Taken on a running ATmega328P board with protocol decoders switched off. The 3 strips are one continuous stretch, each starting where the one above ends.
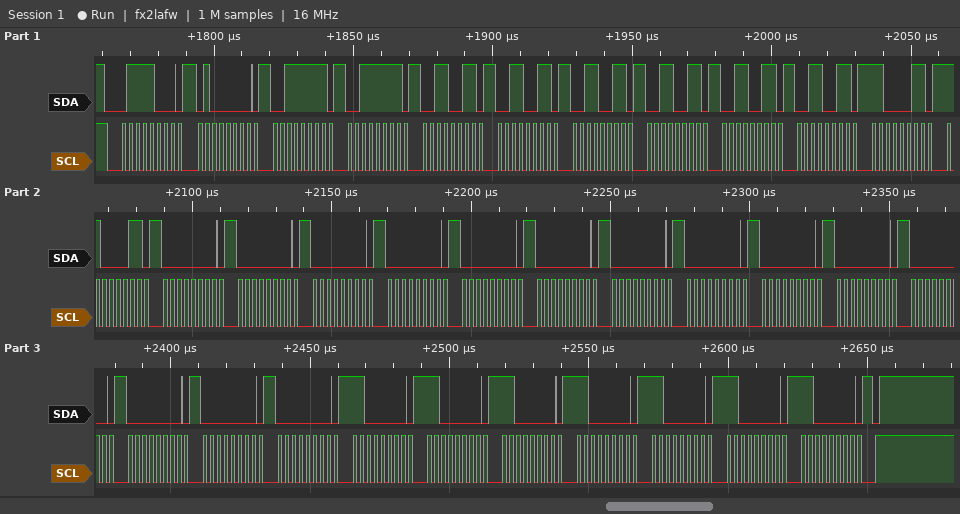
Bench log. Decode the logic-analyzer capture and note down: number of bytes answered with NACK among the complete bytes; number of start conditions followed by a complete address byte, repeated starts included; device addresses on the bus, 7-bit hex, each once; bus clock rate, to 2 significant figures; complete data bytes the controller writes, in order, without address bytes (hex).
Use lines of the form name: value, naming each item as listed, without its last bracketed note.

number of bytes answered with NACK among the complete bytes: 0
number of start conditions followed by a complete address byte, repeated starts included: 1
device addresses on the bus, 7-bit hex, each once: 0x3C
bus clock rate, to 2 significant figures: 400 kHz
complete data bytes the controller writes, in order, without address bytes: 40 3F 3F 33 33 33 33 33 33 C3 C3 00 00 00 00 00 00 00 00 00 00 00 00 00 00 C0 C0 C0 C0 C0 C0 C0
